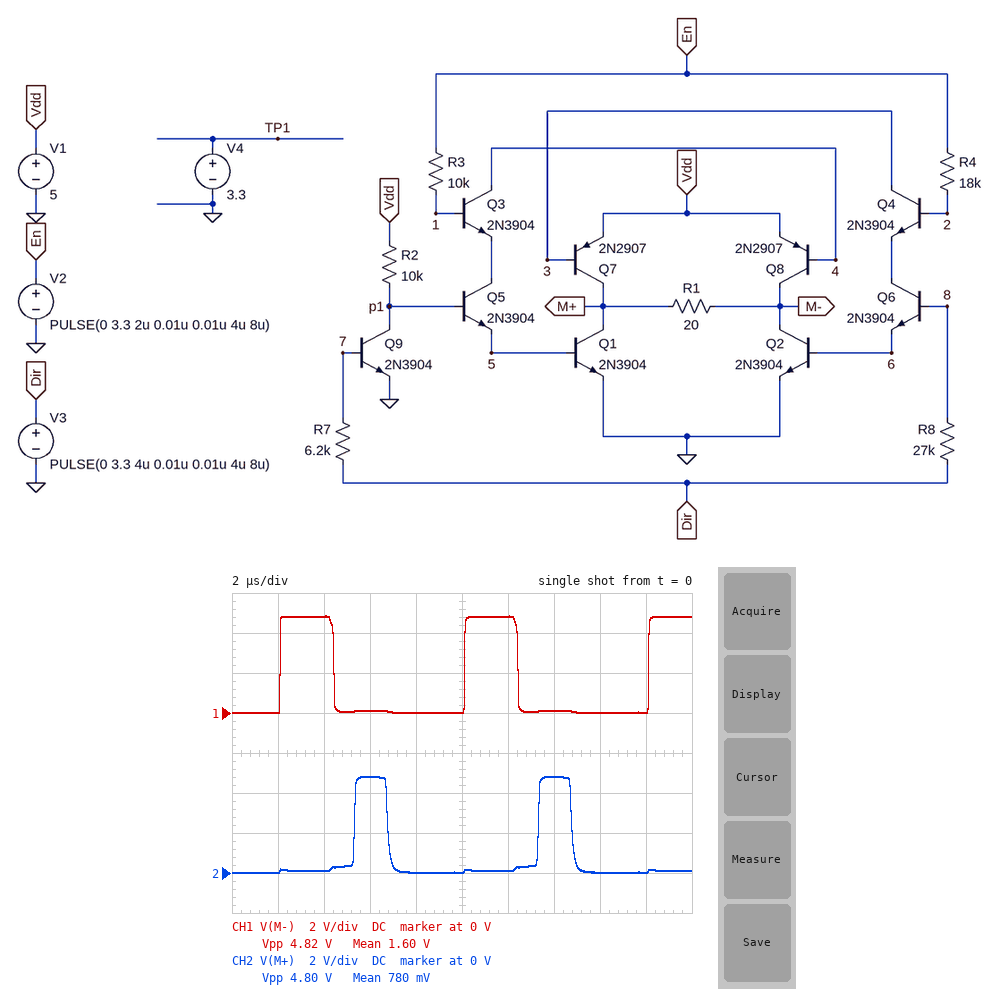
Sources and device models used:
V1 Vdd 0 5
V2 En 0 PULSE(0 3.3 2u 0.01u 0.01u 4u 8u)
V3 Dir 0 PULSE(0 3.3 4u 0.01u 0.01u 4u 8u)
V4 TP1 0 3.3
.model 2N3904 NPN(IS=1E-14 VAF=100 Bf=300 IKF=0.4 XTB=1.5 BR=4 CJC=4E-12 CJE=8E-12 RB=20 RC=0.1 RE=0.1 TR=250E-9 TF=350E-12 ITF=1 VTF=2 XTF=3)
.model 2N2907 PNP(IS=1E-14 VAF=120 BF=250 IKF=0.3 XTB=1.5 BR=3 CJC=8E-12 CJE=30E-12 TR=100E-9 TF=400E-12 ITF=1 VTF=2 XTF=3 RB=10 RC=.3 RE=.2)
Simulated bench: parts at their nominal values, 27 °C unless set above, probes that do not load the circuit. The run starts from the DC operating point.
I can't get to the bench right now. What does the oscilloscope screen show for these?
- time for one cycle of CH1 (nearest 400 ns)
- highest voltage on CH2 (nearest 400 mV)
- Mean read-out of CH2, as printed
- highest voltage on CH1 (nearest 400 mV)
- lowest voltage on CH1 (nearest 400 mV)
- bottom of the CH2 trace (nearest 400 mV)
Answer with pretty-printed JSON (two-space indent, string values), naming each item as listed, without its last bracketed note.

{
  "time for one cycle of CH1": "8.0 µs",
  "highest voltage on CH2": "4.8 V",
  "Mean read-out of CH2, as printed": "780 mV",
  "highest voltage on CH1": "4.8 V",
  "lowest voltage on CH1": "0 V",
  "bottom of the CH2 trace": "0 V"
}
